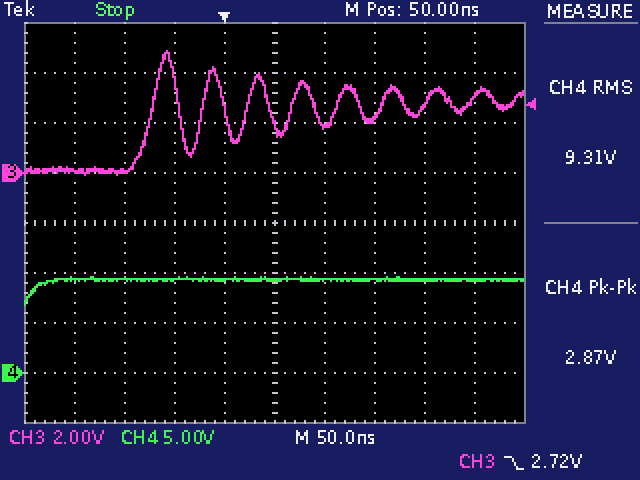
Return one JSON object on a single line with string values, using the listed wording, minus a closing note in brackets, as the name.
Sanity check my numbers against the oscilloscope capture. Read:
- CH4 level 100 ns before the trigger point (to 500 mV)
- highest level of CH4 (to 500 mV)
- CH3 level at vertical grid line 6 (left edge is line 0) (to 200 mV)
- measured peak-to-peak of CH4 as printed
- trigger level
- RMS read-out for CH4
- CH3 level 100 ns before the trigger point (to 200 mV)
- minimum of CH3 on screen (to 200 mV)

{"CH4 level 100 ns before the trigger point": "9.5 V", "highest level of CH4": "9.5 V", "CH3 level at vertical grid line 6 (left edge is line 0)": "1.8 V", "measured peak-to-peak of CH4 as printed": "2.87 V", "trigger level": "2.72 V", "RMS read-out for CH4": "9.31 V", "CH3 level 100 ns before the trigger point": "0.0 V", "minimum of CH3 on screen": "0.0 V"}
